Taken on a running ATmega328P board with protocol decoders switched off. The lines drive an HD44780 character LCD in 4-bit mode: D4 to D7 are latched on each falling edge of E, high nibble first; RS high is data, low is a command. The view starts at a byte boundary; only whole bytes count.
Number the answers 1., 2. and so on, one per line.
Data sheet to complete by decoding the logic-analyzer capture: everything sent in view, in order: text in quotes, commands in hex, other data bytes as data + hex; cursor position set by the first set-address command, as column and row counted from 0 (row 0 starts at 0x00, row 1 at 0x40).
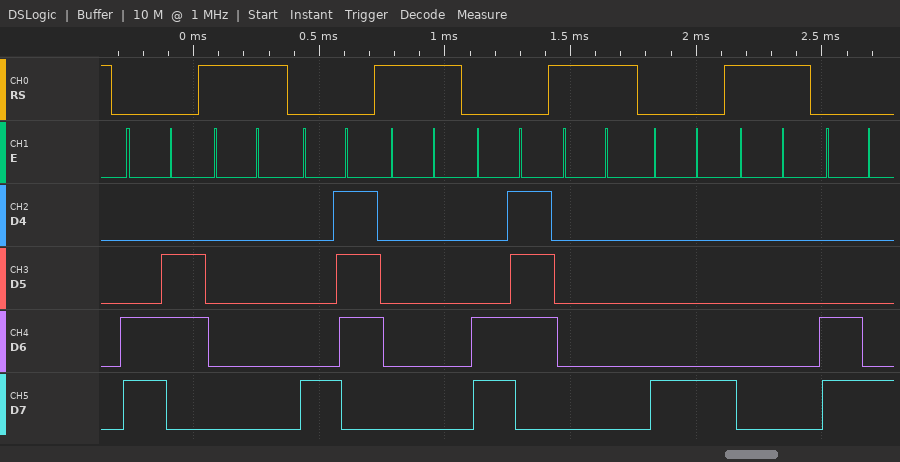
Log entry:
1. 0xC6 data 00 0x87 data 00 0xC7 data 00 0x88 data 00 0xC8
2. column 6, row 1
